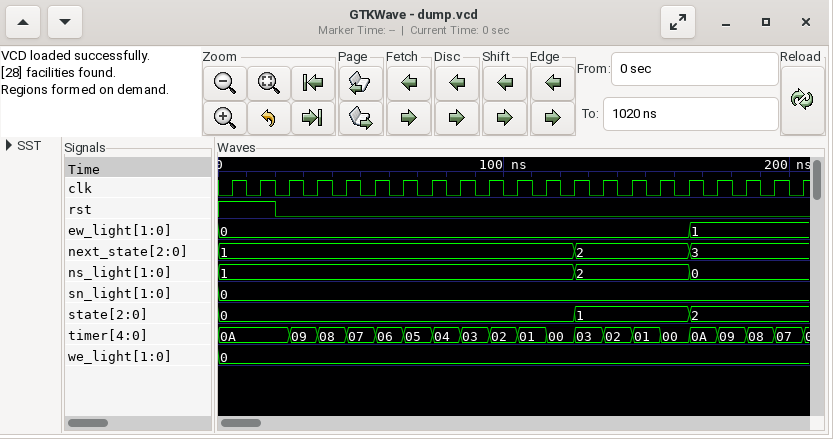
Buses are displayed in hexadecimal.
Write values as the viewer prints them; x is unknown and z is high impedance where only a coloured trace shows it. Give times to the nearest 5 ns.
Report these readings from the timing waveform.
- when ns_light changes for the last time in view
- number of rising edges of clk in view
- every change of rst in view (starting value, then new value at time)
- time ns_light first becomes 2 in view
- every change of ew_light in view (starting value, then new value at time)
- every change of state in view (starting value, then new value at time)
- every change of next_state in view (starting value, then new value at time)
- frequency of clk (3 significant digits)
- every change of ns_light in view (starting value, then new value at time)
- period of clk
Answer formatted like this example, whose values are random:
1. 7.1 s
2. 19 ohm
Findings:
1. 165 ns
2. 21
3. 1, 0 at 20 ns
4. 125 ns
5. 0, 1 at 165 ns
6. 0, 1 at 125 ns, 2 at 165 ns
7. 1, 2 at 125 ns, 3 at 165 ns
8. 100 MHz
9. 1, 2 at 125 ns, 0 at 165 ns
10. 10 ns
